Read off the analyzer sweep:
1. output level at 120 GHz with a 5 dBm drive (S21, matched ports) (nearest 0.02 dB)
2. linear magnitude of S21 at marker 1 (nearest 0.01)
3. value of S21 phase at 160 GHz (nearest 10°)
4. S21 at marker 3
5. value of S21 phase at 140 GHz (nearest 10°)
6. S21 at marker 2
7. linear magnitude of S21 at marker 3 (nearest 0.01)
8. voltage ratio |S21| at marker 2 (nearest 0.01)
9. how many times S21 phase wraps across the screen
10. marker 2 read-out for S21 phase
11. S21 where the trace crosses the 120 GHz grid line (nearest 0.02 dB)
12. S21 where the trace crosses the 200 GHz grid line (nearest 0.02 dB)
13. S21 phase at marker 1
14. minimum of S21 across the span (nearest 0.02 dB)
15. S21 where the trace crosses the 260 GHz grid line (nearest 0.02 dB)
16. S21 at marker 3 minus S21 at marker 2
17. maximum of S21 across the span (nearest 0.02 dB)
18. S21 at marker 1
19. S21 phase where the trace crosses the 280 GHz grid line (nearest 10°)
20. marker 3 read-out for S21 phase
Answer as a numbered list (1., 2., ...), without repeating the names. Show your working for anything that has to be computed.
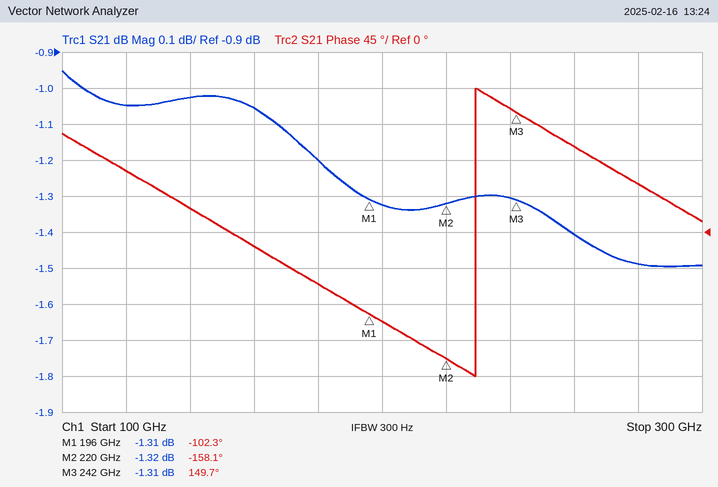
1. 5 dBm + (-1.04 dB) = 3.96 dBm
2. 10^(-1.31/20) ≈ 0.86
3. -20°
4. -1.31 dB
5. 30°
6. -1.32 dB
7. 10^(-1.31/20) ≈ 0.86
8. 10^(-1.32/20) ≈ 0.86
9. 1
10. -158.1°
11. -1.04 dB
12. -1.32 dB
13. -102.3°
14. -1.50 dB
15. -1.40 dB
16. -1.31 − (-1.32) = 0.01 dB
17. -0.96 dB
18. -1.31 dB
19. 60°
20. 149.7°
